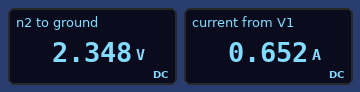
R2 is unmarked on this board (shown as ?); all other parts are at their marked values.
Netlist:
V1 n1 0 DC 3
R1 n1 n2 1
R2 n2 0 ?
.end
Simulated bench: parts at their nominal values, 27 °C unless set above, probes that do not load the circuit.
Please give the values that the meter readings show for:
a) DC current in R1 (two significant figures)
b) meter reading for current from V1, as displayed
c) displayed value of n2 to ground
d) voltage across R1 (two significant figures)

650 mA
0.652 A
2.348 V
650 mV
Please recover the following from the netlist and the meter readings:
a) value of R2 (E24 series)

3.6 Ω
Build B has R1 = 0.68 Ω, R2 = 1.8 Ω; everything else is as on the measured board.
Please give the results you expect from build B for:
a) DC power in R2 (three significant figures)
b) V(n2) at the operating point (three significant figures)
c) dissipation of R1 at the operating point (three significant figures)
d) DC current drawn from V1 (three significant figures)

2.63 W
2.18 V
995 mW
1.21 A
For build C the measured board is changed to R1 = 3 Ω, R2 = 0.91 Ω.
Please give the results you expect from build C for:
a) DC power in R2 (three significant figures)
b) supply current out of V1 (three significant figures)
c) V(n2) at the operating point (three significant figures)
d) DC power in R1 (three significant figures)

536 mW
767 mA
698 mV
1.77 W
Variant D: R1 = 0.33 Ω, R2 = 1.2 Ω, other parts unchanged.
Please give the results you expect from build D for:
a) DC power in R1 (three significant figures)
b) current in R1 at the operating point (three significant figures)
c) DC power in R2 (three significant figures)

1.27 W
1.96 A
4.61 W
